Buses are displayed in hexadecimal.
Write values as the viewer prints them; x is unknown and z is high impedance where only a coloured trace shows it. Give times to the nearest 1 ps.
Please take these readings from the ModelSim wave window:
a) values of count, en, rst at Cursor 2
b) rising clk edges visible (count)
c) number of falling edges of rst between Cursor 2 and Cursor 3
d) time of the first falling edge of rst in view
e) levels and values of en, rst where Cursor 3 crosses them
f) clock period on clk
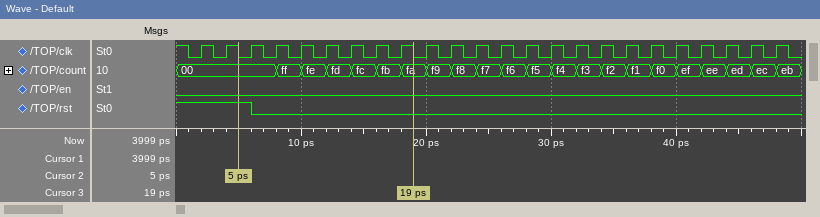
count=00, en=0, rst=1
24
1
6 ps
en=0, rst=0
2 ps
